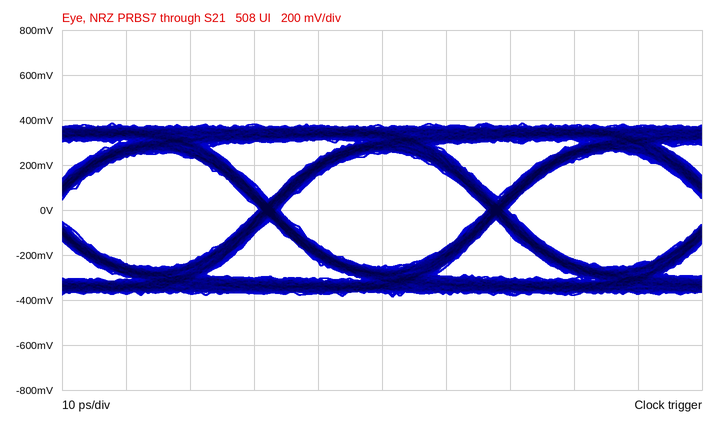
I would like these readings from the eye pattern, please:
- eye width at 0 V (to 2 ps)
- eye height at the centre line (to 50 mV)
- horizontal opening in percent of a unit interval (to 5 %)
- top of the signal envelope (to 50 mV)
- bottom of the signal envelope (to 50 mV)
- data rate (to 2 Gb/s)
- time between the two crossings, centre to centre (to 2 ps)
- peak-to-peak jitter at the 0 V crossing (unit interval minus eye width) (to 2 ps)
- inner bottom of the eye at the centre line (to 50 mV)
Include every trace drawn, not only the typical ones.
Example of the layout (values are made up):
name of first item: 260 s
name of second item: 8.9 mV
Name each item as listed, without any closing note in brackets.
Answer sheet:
eye width at 0 V: 32 ps
eye height at the centre line: 500 mV
horizontal opening in percent of a unit interval: 90 %
top of the signal envelope: 400 mV
bottom of the signal envelope: -400 mV
data rate: 28 Gb/s
time between the two crossings, centre to centre: 36 ps
peak-to-peak jitter at the 0 V crossing (unit interval minus eye width): 4 ps
inner bottom of the eye at the centre line: -250 mV
